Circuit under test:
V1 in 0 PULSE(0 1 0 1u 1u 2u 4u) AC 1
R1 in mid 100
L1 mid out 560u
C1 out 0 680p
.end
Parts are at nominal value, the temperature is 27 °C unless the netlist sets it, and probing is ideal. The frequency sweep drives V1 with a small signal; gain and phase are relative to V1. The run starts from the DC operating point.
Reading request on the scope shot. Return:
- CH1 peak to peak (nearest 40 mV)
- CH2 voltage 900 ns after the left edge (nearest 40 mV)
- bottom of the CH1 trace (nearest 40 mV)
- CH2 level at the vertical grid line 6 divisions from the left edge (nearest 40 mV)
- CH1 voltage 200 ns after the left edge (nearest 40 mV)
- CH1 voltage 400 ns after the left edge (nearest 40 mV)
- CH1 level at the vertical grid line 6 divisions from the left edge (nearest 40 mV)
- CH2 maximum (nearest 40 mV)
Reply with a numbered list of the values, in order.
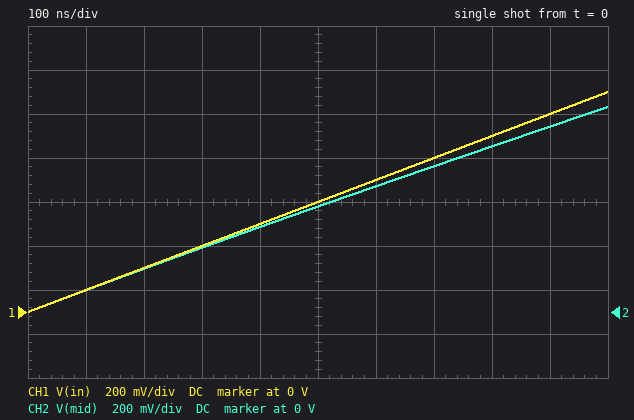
1. 1.00 V
2. 840 mV
3. 0 V
4. 560 mV
5. 200 mV
6. 400 mV
7. 600 mV
8. 920 mV
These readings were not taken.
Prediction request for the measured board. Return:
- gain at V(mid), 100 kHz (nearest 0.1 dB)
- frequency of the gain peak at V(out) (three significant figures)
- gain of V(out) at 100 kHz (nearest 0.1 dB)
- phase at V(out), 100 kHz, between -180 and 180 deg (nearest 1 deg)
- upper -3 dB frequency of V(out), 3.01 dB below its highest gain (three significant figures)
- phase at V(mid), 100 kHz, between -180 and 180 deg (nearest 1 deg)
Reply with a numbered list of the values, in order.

1. 0 dB
2. 257 kHz
3. 1.4 dB
4. -3 deg
5. 271 kHz
6. -3 deg
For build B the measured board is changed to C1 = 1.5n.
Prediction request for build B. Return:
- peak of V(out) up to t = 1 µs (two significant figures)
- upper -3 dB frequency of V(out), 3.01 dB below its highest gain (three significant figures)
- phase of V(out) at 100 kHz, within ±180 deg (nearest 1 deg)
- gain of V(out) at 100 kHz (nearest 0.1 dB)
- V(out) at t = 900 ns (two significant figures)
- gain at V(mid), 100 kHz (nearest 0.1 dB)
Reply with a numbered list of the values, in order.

1. 180 mV
2. 186 kHz
3. -8 deg
4. 3.4 dB
5. 130 mV
6. -0.1 dB
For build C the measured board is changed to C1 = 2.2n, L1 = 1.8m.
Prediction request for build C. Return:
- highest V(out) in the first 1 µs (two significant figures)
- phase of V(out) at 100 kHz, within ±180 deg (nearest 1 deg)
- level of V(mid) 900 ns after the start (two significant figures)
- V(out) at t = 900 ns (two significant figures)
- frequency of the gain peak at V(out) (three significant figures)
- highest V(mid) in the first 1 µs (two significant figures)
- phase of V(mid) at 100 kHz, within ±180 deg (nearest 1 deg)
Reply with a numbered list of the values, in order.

1. 41 mV
2. -166 deg
3. 880 mV
4. 30 mV
5. 79.7 kHz
6. 970 mV
7. 14 deg
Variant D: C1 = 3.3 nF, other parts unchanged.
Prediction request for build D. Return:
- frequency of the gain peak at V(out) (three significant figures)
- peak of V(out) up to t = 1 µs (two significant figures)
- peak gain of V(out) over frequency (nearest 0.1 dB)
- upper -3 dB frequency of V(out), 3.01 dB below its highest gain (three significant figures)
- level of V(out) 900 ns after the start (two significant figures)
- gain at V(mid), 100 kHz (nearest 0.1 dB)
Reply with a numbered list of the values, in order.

1. 115 kHz
2. 84 mV
3. 12.4 dB
4. 129 kHz
5. 62 mV
6. -2.0 dB
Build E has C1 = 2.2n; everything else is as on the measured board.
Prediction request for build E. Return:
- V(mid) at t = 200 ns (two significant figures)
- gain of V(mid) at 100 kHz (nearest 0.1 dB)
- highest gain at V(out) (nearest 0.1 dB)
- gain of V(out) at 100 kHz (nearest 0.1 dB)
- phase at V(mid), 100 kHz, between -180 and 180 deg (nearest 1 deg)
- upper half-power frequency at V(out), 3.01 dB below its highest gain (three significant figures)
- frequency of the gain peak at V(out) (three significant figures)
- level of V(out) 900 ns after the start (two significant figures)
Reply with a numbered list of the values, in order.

1. 200 mV
2. -0.3 dB
3. 14.1 dB
4. 5.5 dB
5. -15 deg
6. 156 kHz
7. 142 kHz
8. 92 mV
